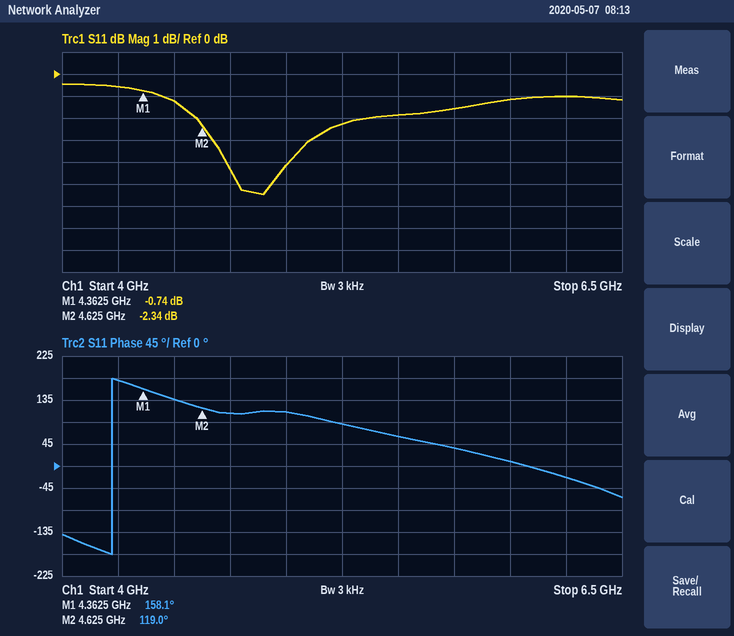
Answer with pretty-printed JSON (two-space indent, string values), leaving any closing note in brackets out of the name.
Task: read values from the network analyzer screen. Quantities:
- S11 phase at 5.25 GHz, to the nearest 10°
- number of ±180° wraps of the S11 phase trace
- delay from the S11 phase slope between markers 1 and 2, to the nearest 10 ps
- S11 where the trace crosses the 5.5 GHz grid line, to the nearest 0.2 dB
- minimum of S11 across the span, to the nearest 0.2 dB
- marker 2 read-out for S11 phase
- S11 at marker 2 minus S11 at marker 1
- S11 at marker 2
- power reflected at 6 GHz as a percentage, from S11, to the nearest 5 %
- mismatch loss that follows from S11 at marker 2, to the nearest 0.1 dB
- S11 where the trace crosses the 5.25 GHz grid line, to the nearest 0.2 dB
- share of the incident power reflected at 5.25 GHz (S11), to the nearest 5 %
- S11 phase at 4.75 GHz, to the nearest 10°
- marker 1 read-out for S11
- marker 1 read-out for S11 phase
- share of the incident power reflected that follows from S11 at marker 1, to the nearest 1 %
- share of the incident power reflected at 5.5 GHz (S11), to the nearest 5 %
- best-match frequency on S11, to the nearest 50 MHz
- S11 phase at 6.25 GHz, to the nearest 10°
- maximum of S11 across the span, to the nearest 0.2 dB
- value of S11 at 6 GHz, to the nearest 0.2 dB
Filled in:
{
  "S11 phase at 5.25 GHz, to the nearest 10°": "90°",
  "number of ±180° wraps of the S11 phase trace": "1",
  "delay from the S11 phase slope between markers 1 and 2, to the nearest 10 ps": "410 ps",
  "S11 where the trace crosses the 5.5 GHz grid line, to the nearest 0.2 dB": "-1.8 dB",
  "minimum of S11 across the span, to the nearest 0.2 dB": "-5.4 dB",
  "marker 2 read-out for S11 phase": "119.0°",
  "S11 at marker 2 minus S11 at marker 1": "-1.60 dB",
  "S11 at marker 2": "-2.34 dB",
  "power reflected at 6 GHz as a percentage, from S11, to the nearest 5 %": "75 %",
  "mismatch loss that follows from S11 at marker 2, to the nearest 0.1 dB": "3.8 dB",
  "S11 where the trace crosses the 5.25 GHz grid line, to the nearest 0.2 dB": "-2.2 dB",
  "share of the incident power reflected at 5.25 GHz (S11), to the nearest 5 %": "60 %",
  "S11 phase at 4.75 GHz, to the nearest 10°": "110°",
  "marker 1 read-out for S11": "-0.74 dB",
  "marker 1 read-out for S11 phase": "158.1°",
  "share of the incident power reflected that follows from S11 at marker 1, to the nearest 1 %": "84 %",
  "share of the incident power reflected at 5.5 GHz (S11), to the nearest 5 %": "65 %",
  "best-match frequency on S11, to the nearest 50 MHz": "4.90 GHz",
  "S11 phase at 6.25 GHz, to the nearest 10°": "-20°",
  "maximum of S11 across the span, to the nearest 0.2 dB": "-0.4 dB",
  "value of S11 at 6 GHz, to the nearest 0.2 dB": "-1.2 dB"
}
